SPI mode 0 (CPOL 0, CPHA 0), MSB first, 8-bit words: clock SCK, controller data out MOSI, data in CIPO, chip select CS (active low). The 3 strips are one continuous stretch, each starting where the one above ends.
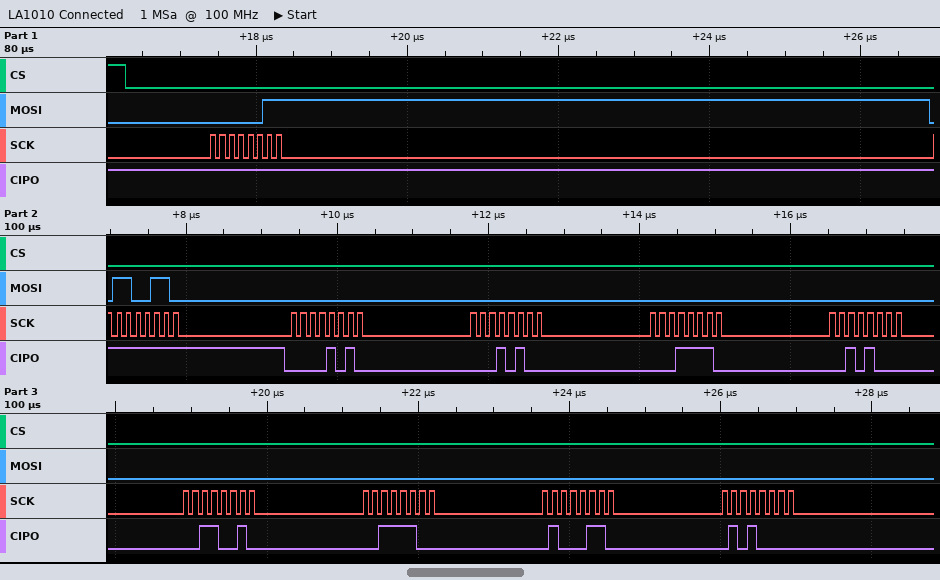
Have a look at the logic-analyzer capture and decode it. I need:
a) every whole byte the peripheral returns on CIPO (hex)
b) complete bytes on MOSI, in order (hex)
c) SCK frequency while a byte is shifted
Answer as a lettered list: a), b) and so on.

a) FF FF 0A 14 1E 28 32 3C 46 50
b) 03 66 00 00 00 00 00 00 00 00
c) 8 MHz
